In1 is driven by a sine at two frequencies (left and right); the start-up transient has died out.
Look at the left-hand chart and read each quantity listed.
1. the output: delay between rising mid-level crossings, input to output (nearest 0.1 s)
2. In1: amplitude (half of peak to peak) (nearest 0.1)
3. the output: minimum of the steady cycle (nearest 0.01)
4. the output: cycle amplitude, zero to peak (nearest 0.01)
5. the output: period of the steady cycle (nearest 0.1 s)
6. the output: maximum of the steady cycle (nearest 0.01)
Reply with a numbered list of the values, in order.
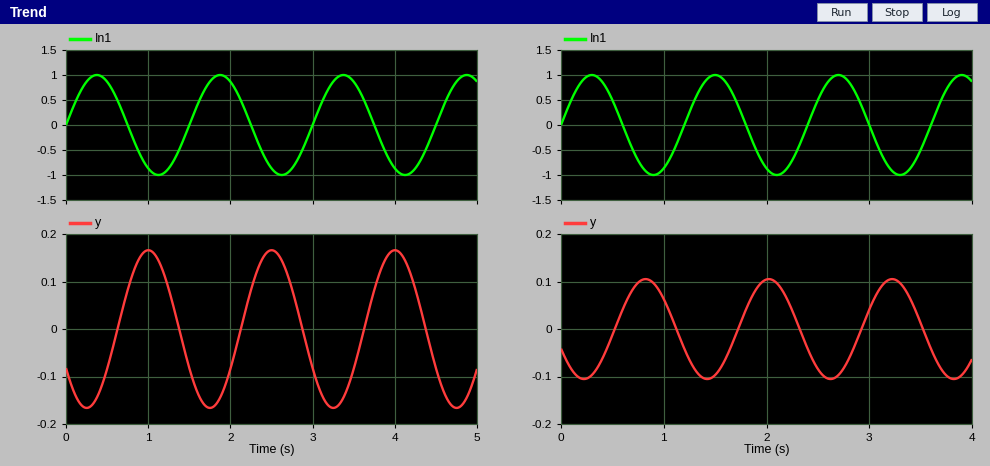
1. 0.6 s
2. 1.0
3. -0.17
4. 0.17
5. 1.5 s
6. 0.17
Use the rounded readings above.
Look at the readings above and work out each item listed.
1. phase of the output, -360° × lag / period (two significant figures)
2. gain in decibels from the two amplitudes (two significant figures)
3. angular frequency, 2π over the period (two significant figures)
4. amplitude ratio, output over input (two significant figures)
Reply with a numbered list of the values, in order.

1. -140°
2. -15 dB
3. 4.2 rad/s
4. 0.17
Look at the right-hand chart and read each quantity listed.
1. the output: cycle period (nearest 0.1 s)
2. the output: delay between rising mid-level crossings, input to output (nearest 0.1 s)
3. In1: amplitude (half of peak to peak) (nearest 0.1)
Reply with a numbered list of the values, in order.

1. 1.2 s
2. 0.5 s
3. 1.0
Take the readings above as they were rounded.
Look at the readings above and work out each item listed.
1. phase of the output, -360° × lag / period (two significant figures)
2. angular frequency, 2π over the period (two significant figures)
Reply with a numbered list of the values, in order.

1. -150°
2. 5.2 rad/s
